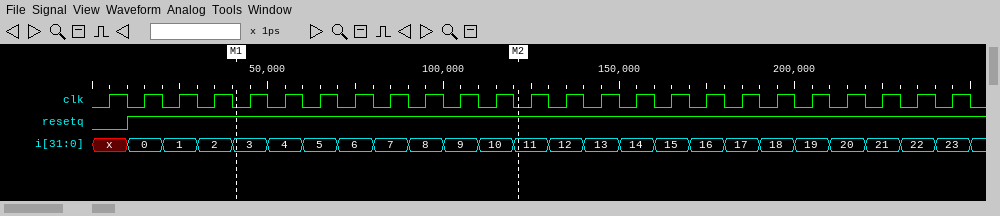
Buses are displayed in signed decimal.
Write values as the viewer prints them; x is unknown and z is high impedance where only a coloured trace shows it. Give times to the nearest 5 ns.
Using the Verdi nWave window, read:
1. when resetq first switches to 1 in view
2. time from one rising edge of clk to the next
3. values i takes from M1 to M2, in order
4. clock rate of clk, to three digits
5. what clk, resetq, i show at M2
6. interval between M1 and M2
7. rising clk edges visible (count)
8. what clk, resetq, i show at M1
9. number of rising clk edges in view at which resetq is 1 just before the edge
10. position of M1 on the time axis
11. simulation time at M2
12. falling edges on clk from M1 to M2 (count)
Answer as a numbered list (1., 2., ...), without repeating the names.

1. 10 ns
2. 10 ns
3. 3, 4, 5, 6, 7, 8, 9, 10, 11
4. 100 MHz
5. clk=0, resetq=1, i=11
6. 80 ns
7. 25
8. clk=0, resetq=1, i=3
9. 24
10. 40 ns
11. 120 ns
12. 8
